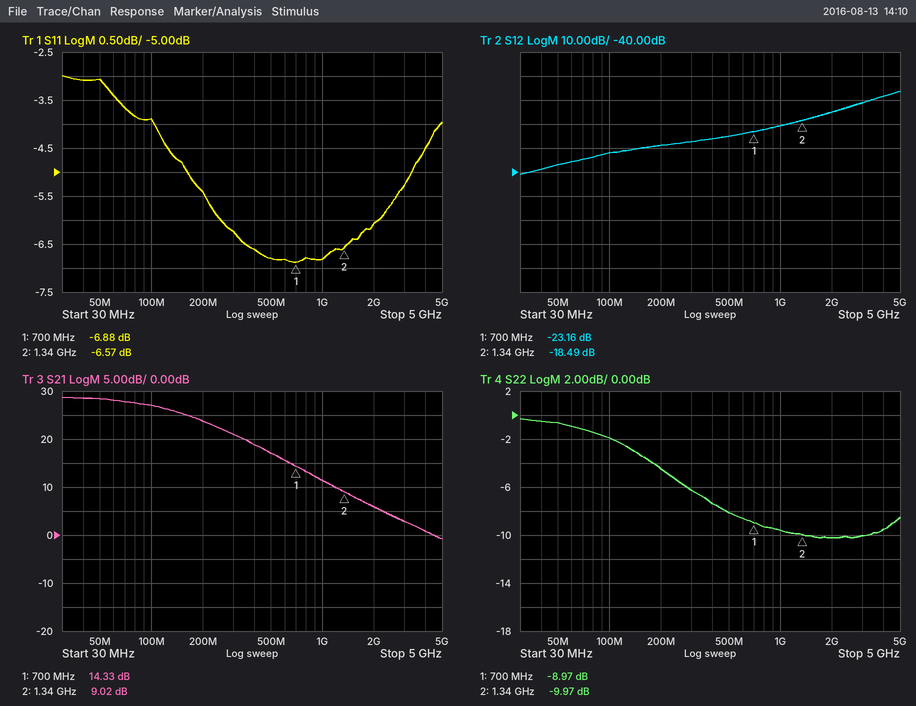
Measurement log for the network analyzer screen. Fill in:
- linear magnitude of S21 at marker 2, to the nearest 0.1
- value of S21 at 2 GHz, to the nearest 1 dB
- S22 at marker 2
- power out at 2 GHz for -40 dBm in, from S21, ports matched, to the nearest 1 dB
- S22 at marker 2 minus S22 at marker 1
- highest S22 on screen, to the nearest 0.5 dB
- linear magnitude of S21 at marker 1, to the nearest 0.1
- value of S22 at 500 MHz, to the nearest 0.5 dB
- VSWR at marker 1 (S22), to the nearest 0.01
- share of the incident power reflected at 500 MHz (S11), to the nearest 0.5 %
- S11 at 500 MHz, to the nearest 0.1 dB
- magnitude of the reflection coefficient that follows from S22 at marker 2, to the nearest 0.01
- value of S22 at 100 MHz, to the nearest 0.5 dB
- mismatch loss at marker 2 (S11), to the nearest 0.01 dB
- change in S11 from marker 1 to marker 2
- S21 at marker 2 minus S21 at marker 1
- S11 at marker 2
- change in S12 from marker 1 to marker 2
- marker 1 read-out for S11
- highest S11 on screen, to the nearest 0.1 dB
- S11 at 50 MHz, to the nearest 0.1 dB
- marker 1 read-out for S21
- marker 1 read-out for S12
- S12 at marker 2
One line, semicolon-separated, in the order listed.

2.8; 6 dB; -9.97 dB; -34 dBm; -1.00 dB; -0.5 dB; 5.2; -8.0 dB; 2.11; 21.0 %; -6.8 dB; 0.32; -2.0 dB; 1.08 dB; 0.31 dB; -5.31 dB; -6.57 dB; 4.67 dB; -6.88 dB; -3.0 dB; -3.1 dB; 14.33 dB; -23.16 dB; -18.49 dB
